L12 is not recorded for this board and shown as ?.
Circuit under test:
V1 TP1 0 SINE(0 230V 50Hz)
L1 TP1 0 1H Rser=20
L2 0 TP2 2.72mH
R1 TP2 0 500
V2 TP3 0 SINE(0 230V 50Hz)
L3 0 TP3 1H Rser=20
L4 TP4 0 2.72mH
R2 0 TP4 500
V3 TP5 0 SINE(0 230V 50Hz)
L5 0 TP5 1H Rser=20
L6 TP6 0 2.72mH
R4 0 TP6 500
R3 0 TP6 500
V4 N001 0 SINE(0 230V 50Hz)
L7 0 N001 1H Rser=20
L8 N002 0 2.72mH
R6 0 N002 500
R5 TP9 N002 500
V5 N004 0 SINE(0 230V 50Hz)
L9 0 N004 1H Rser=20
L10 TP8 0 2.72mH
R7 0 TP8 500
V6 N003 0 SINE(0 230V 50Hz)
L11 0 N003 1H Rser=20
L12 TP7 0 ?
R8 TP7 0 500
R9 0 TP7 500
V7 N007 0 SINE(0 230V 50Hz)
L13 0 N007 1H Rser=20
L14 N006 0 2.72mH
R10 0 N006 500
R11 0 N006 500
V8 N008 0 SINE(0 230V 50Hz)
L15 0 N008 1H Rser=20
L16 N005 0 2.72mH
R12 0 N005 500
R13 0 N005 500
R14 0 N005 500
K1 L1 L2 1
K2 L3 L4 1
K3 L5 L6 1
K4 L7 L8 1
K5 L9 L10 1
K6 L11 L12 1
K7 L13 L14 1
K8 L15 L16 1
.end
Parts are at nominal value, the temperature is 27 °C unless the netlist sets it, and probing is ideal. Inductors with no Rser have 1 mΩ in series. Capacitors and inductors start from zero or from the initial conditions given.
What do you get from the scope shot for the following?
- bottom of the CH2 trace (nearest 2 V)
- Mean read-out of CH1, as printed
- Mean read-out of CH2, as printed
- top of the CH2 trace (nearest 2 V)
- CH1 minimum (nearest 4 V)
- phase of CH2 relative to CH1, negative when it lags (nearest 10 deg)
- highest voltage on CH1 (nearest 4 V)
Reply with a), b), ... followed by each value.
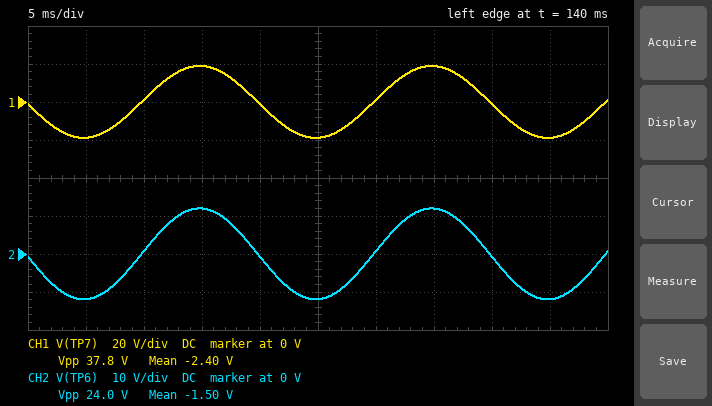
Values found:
a) -12 V
b) -2.40 V
c) -1.50 V
d) 12 V
e) -20 V
f) 0 deg
g) 20 V
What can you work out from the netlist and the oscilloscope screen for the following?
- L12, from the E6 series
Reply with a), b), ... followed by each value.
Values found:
a) 6.8 mH
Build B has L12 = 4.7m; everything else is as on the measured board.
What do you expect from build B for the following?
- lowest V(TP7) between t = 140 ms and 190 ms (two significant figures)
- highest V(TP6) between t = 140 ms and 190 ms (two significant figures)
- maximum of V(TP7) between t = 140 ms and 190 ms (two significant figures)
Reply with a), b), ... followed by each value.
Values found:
a) -16 V
b) 12 V
c) 16 V
